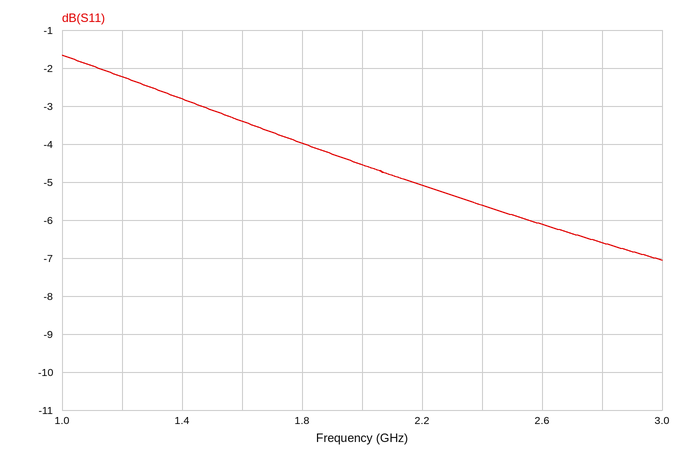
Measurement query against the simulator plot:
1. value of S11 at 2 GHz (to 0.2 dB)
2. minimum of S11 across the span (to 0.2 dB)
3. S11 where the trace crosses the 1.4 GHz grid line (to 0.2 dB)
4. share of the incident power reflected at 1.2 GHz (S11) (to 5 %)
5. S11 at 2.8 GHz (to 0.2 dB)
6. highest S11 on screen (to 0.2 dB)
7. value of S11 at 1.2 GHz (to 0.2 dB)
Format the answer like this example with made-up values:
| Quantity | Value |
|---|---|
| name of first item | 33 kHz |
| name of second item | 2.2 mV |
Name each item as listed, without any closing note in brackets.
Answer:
| Quantity | Value |
|---|---|
| value of S11 at 2 GHz | -4.6 dB |
| minimum of S11 across the span | -7.0 dB |
| S11 where the trace crosses the 1.4 GHz grid line | -2.8 dB |
| share of the incident power reflected at 1.2 GHz (S11) | 60 % |
| S11 at 2.8 GHz | -6.6 dB |
| highest S11 on screen | -1.6 dB |
| value of S11 at 1.2 GHz | -2.2 dB |
